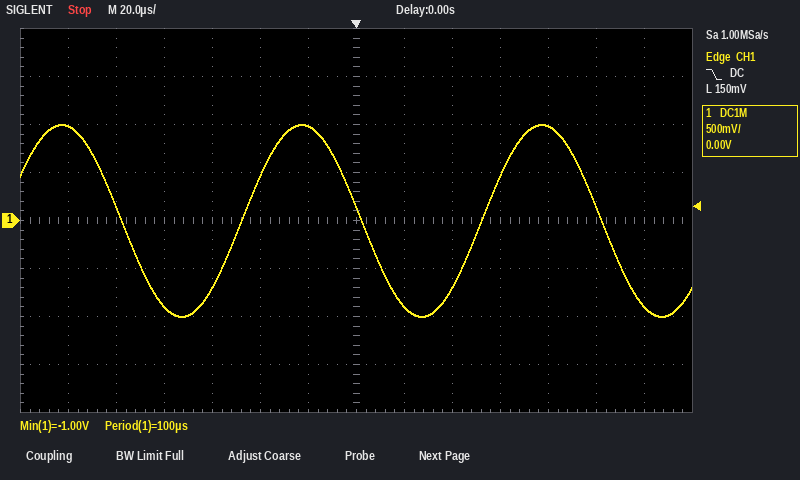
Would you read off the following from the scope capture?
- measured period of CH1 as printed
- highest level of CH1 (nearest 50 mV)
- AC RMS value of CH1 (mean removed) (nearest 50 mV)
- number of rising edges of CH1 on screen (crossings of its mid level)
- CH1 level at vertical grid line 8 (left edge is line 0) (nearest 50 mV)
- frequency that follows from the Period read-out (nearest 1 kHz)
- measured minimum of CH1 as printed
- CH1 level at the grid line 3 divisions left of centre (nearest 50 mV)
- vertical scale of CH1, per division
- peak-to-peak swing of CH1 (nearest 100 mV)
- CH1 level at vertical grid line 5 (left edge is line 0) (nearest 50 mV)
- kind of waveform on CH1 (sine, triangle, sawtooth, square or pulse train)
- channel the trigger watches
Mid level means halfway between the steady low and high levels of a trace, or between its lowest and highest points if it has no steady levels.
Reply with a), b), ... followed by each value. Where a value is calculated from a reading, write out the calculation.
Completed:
a) 100 µs
b) 1.00 V
c) 2.00 V / (2√2) ≈ 707 mV, so 700 mV to the nearest 50 mV
d) 2
e) -900 mV
f) 1 / 100 µs ≈ 10 kHz
g) -1.00 V
h) -700 mV
i) 500 mV
j) 2.00 V
k) 450 mV
l) sine
m) CH1
